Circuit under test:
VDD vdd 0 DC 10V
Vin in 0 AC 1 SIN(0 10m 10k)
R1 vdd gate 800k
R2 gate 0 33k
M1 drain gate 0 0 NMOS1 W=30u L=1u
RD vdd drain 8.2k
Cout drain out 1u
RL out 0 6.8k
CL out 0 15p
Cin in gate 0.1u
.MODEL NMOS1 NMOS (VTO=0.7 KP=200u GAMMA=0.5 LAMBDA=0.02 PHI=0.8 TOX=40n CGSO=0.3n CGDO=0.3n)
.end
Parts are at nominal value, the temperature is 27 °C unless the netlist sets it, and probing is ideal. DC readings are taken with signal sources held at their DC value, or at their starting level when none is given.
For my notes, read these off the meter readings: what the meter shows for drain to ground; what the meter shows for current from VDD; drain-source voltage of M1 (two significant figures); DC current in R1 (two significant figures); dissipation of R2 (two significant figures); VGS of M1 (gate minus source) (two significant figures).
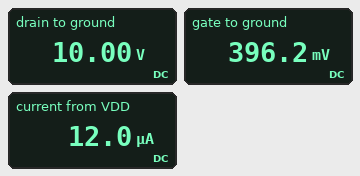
10.00 V
12.0 µA
10 V
12 µA
4.8 µW
400 mV
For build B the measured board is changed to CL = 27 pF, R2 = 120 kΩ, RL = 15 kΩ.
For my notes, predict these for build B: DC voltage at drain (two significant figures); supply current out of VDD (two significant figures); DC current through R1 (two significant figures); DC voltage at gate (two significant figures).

860 mV
1.1 mA
11 µA
1.3 V
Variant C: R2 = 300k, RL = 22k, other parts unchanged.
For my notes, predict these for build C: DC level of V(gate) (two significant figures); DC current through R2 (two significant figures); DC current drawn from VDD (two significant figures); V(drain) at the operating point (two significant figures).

2.7 V
9.1 µA
1.2 mA
100 mV
